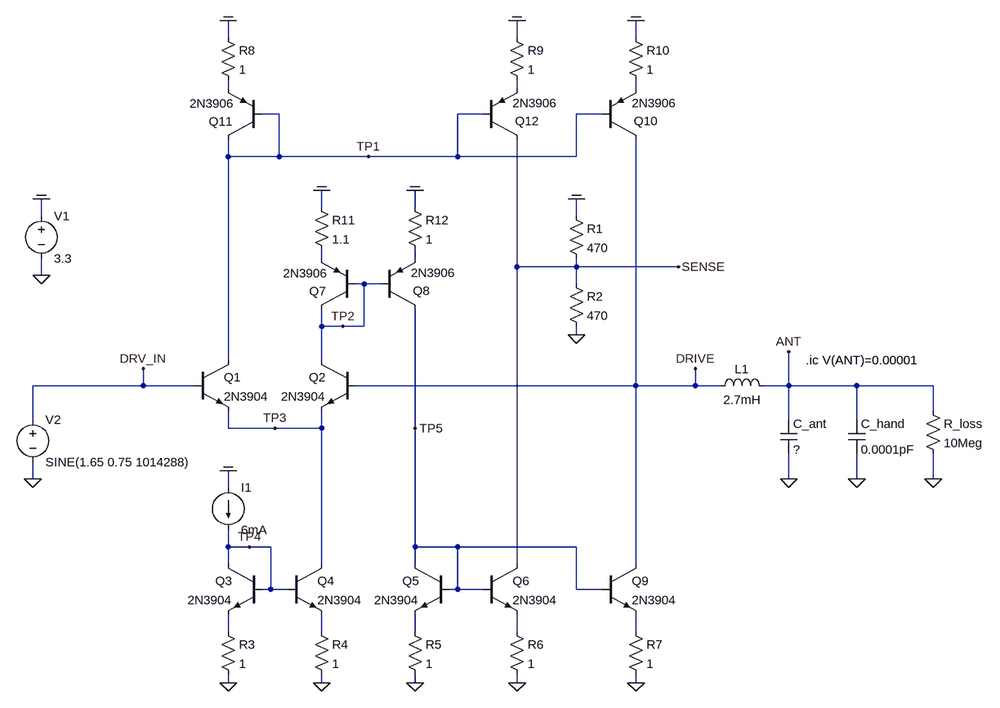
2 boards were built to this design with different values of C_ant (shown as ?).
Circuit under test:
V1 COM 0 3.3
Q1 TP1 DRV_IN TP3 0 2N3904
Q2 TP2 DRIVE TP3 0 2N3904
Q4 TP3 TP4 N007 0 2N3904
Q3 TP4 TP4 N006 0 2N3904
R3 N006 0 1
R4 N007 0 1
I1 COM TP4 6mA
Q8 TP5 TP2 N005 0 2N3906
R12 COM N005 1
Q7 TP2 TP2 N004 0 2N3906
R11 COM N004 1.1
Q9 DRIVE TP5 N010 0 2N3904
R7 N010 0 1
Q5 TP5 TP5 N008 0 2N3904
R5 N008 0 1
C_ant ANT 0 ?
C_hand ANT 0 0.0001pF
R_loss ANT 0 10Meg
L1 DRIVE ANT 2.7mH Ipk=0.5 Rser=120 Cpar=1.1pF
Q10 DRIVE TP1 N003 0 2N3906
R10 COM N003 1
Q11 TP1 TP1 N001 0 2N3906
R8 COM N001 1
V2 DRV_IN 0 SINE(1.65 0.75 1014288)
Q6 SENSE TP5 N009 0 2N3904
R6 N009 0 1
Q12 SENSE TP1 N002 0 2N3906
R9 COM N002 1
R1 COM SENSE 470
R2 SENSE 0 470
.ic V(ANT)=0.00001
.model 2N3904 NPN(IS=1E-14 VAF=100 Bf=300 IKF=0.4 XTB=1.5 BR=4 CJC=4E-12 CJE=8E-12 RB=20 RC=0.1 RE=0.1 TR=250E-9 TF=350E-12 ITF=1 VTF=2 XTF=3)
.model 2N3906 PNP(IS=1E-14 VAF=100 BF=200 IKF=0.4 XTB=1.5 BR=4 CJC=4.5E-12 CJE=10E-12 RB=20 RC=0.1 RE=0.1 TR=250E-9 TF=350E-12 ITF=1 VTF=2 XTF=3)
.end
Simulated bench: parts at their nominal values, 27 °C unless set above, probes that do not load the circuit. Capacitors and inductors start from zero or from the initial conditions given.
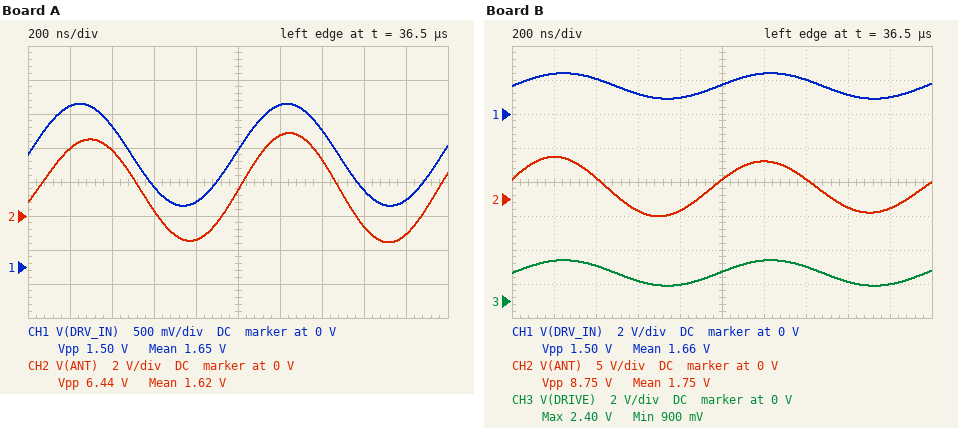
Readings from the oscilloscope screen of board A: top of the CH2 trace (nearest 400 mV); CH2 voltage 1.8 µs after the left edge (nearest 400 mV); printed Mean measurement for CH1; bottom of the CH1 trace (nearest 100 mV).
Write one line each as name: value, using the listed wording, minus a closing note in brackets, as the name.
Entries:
top of the CH2 trace: 4.8 V
CH2 voltage 1.8 µs after the left edge: -1.2 V
printed Mean measurement for CH1: 1.65 V
bottom of the CH1 trace: 900 mV
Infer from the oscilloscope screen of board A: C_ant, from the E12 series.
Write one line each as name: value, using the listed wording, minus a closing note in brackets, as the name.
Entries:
C_ant, from the E12 series: 5.6 pF
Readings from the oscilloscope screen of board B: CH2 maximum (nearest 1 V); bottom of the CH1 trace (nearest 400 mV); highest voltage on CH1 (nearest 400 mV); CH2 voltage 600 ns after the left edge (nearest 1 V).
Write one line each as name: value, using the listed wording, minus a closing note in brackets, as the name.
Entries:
CH2 maximum: 6 V
bottom of the CH1 trace: 800 mV
highest voltage on CH1: 2.4 V
CH2 voltage 600 ns after the left edge: -2 V
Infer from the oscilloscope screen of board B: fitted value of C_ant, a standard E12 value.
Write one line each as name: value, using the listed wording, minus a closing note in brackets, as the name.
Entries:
fitted value of C_ant, a standard E12 value: 6.8 pF
